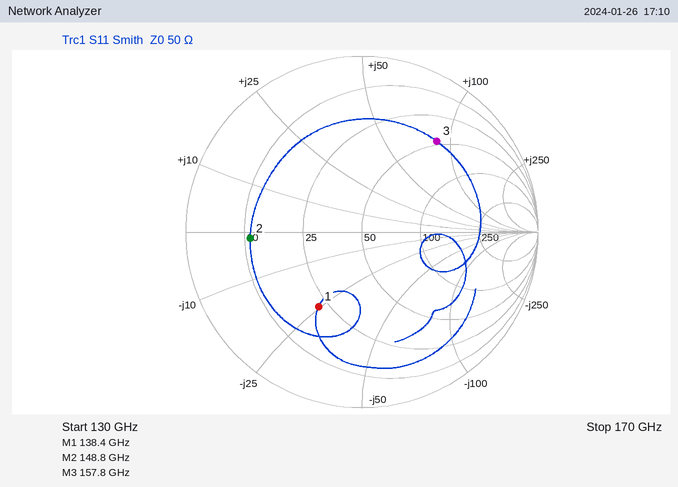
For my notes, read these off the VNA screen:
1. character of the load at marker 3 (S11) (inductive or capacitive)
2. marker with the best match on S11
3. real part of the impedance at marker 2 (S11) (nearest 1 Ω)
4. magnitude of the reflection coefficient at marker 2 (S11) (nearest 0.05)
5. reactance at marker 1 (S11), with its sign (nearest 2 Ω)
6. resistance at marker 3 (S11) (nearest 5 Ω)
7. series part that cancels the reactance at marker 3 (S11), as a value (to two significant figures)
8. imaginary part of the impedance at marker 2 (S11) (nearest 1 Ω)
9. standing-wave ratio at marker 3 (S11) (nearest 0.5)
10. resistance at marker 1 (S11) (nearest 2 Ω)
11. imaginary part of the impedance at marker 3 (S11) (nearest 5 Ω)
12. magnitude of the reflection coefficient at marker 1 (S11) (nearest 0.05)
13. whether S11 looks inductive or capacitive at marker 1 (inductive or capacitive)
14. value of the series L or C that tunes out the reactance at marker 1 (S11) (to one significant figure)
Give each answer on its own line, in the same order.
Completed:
inductive
marker 1
11 Ω
0.65
-24 Ω
45 Ω
12 fF
-1 Ω
5.0
22 Ω
+85 Ω
0.50
capacitive
30 pH
